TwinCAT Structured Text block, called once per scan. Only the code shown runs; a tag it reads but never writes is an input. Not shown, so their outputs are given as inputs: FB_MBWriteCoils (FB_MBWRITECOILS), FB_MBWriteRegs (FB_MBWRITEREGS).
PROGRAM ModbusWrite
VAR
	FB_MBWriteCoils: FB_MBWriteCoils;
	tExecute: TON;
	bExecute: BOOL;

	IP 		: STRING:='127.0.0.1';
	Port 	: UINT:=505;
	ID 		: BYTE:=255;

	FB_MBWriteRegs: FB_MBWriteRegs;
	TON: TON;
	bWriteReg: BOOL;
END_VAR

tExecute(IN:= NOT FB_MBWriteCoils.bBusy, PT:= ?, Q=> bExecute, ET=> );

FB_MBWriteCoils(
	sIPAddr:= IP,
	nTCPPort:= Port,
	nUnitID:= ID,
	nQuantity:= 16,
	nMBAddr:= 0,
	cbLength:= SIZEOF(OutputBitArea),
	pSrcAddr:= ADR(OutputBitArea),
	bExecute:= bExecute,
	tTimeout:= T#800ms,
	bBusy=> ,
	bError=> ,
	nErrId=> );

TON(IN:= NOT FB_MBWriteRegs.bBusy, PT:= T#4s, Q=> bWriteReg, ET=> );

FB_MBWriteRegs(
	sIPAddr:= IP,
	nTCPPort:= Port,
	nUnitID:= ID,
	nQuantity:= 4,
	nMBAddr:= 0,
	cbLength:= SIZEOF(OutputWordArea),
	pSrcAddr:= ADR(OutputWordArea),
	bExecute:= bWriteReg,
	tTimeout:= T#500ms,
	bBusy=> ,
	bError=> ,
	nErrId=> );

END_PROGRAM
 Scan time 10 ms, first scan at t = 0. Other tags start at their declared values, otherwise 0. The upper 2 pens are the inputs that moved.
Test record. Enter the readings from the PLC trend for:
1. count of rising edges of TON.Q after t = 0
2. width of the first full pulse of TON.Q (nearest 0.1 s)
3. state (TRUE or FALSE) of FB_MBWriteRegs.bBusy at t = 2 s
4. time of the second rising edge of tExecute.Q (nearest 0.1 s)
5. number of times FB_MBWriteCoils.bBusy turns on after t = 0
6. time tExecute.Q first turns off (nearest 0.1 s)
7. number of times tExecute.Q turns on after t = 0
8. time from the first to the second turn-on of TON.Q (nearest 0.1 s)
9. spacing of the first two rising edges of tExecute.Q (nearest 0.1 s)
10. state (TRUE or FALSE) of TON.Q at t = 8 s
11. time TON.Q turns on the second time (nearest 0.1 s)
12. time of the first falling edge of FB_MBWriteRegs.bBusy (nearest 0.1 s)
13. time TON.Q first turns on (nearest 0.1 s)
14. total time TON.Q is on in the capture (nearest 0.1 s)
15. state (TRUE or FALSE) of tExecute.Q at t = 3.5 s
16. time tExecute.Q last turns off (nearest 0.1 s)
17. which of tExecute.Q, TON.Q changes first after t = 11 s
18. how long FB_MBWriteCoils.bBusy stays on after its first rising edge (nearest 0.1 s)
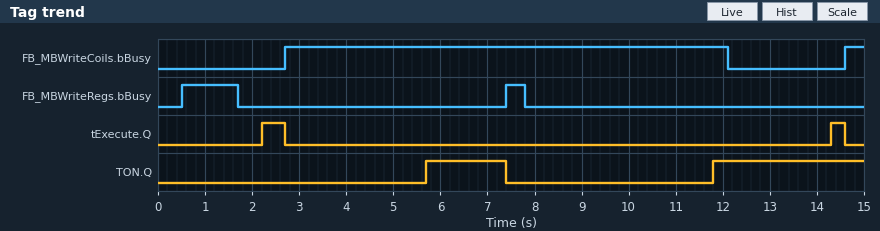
2
1.7 s
FALSE
14.3 s
2
2.7 s
2
6.1 s
12.1 s
FALSE
11.8 s
1.7 s
5.7 s
4.9 s
FALSE
14.6 s
TON.Q
9.4 s
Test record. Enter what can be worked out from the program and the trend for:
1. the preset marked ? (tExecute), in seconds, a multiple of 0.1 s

2.2 s
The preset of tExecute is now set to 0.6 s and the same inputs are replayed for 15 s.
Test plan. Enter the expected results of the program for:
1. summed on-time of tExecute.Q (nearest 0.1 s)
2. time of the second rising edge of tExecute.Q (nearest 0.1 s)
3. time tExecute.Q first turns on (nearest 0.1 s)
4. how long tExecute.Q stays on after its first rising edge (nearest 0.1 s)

4.0 s
12.7 s
0.6 s
2.1 s
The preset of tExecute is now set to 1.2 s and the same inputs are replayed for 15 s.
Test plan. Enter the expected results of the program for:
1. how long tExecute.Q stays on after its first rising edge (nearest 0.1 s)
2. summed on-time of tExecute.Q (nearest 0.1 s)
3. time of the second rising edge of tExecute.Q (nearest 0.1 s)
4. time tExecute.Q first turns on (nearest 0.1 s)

1.5 s
2.8 s
13.3 s
1.2 s
